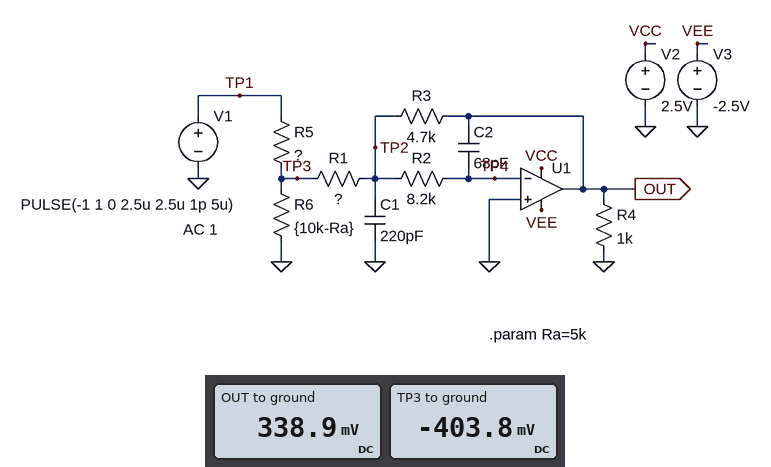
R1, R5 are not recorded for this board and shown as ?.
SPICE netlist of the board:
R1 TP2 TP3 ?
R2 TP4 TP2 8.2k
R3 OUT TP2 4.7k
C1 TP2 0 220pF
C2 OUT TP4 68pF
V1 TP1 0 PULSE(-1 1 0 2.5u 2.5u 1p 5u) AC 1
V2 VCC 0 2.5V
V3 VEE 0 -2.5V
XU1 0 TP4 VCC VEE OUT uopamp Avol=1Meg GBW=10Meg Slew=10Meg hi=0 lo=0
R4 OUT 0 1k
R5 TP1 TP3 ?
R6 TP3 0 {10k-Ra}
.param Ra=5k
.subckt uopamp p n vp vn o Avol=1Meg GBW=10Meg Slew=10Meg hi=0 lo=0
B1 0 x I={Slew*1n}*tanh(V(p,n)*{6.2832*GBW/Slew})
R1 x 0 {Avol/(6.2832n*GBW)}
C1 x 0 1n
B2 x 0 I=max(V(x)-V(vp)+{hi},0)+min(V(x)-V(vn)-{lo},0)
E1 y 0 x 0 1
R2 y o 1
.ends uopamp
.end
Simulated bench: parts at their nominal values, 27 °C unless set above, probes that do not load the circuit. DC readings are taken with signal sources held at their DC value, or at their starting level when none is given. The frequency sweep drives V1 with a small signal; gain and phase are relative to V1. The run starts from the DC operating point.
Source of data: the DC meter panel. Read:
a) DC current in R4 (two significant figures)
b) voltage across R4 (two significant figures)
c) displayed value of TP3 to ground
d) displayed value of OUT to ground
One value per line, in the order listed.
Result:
340 µA
340 mV
-403.8 mV
338.9 mV
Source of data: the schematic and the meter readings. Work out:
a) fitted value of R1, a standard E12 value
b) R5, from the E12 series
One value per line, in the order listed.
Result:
5.6 kΩ
3.9 kΩ
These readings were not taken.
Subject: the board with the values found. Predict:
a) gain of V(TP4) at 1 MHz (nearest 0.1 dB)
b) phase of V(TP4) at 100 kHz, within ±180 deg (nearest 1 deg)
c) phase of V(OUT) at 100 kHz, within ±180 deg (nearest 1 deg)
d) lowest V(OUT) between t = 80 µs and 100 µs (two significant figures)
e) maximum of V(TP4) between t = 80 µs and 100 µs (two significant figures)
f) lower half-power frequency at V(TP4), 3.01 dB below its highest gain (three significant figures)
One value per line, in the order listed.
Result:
-56.9 dB
44 deg
134 deg
-180 mV
3.8 mV
99.7 kHz
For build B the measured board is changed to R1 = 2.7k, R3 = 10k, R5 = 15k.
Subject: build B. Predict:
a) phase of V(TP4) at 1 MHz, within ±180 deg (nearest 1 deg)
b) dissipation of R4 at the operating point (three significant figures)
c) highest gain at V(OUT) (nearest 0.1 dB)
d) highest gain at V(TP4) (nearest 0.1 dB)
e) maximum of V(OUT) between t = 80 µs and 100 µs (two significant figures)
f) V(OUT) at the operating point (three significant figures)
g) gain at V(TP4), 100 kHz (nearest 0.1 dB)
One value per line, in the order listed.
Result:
-80 deg
150 µW
-8.2 dB
-50.7 dB
110 mV
388 mV
-51.3 dB
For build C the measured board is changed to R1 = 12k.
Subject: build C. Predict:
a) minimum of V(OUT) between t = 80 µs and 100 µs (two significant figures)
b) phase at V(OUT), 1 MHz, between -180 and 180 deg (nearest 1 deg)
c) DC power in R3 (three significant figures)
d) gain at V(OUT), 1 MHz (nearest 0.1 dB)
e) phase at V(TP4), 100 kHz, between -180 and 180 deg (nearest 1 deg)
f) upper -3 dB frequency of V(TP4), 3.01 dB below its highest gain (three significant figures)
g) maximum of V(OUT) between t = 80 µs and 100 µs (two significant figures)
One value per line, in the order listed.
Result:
-110 mV
11 deg
7.37 µW
-42.0 dB
48 deg
394 kHz
110 mV
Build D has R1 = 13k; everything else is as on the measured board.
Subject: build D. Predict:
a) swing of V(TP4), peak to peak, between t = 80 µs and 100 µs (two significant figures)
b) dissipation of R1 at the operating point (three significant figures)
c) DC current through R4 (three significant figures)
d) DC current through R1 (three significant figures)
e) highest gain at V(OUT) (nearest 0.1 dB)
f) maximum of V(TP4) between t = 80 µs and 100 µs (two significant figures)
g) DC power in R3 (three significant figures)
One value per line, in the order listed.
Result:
4.4 mV
17.8 µW
174 µA
37.0 µA
-15.2 dB
2.2 mV
6.43 µW
